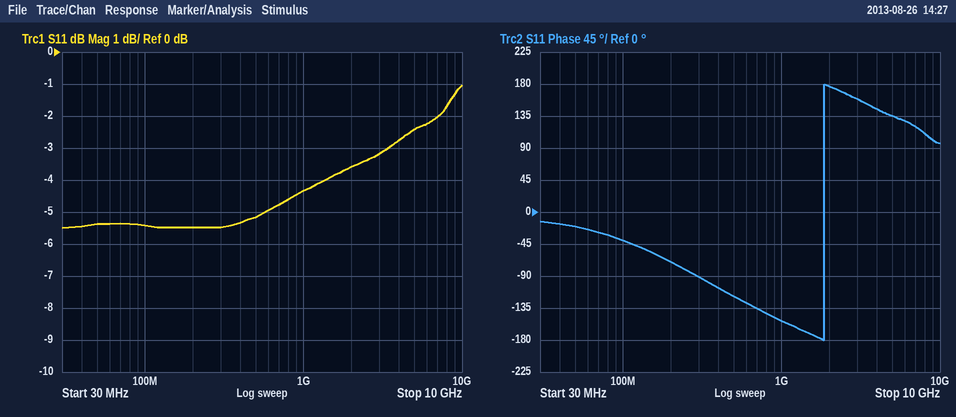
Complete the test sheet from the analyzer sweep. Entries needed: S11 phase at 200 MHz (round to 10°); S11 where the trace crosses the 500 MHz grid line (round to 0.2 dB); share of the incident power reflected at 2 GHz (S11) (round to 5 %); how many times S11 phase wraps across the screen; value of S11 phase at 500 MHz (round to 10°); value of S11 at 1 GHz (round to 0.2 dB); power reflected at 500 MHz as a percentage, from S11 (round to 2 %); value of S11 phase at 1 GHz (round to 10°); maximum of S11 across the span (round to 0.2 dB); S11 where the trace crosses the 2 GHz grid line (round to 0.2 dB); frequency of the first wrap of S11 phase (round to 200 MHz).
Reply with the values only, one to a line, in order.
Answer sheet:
-70°
-5.2 dB
45 %
1
-120°
-4.4 dB
30 %
-150°
-1.0 dB
-3.6 dB
1.8 GHz
